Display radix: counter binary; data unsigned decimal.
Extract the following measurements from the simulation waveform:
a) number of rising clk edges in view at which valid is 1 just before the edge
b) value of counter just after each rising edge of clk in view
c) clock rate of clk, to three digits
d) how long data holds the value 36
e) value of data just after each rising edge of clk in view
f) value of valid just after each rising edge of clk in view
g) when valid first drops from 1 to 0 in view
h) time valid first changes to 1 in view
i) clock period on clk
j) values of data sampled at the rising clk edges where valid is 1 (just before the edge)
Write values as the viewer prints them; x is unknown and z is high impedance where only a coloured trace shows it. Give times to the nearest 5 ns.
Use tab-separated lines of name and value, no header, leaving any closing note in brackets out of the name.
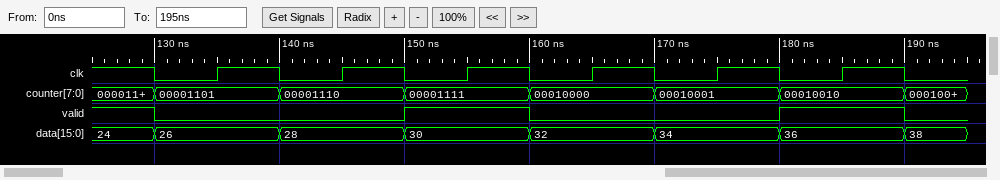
number of rising clk edges in view at which valid is 1 just before the edge	2
value of counter just after each rising edge of clk in view	00001101, 00001110, 00001111, 00010000, 00010001, 00010010
clock rate of clk, to three digits	100 MHz
how long data holds the value 36	10 ns
value of data just after each rising edge of clk in view	26, 28, 30, 32, 34, 36
value of valid just after each rising edge of clk in view	0 0 1 0 0 1
when valid first drops from 1 to 0 in view	130 ns
time valid first changes to 1 in view	150 ns
clock period on clk	10 ns
values of data sampled at the rising clk edges where valid is 1	30, 36
